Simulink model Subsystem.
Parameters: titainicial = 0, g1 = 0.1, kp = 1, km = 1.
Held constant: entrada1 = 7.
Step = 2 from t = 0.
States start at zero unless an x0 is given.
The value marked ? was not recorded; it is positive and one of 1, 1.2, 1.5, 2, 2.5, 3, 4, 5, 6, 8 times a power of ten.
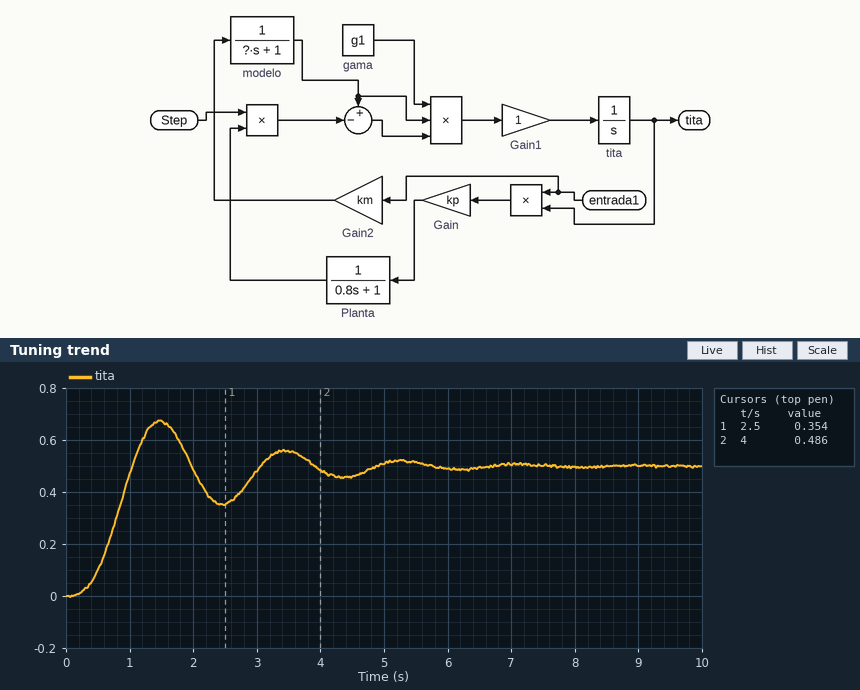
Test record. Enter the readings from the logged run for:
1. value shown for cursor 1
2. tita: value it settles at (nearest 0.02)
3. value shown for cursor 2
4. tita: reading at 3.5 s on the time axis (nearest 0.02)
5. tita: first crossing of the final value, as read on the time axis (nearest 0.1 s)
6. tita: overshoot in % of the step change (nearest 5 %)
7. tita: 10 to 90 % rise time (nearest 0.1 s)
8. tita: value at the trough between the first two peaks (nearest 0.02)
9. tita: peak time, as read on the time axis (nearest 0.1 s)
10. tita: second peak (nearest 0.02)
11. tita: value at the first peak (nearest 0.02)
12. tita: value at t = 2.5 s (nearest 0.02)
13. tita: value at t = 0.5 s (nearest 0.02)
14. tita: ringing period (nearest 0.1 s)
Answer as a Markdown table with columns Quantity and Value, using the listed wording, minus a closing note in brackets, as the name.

| Quantity | Value |
|---|---|
| value shown for cursor 1 | 0.354 |
| tita: value it settles at | 0.50 |
| value shown for cursor 2 | 0.486 |
| tita: reading at 3.5 s on the time axis | 0.56 |
| tita: first crossing of the final value, as read on the time axis | 1.0 s |
| tita: overshoot in % of the step change | 35 % |
| tita: 10 to 90 % rise time | 0.6 s |
| tita: value at the trough between the first two peaks | 0.36 |
| tita: peak time, as read on the time axis | 1.5 s |
| tita: second peak | 0.56 |
| tita: value at the first peak | 0.68 |
| tita: value at t = 2.5 s | 0.36 |
| tita: value at t = 0.5 s | 0.10 |
| tita: ringing period | 2.0 s |
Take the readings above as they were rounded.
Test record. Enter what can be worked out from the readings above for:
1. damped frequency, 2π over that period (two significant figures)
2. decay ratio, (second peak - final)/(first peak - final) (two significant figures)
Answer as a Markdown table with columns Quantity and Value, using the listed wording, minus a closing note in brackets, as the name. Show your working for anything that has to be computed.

| Quantity | Value |
|---|---|
| damped frequency, 2π over that period | 2π / 2 = 3.1 rad/s |
| decay ratio, (second peak - final)/(first peak - final) | (0.56 - 0.5) / (0.68 - 0.5) = 0.33 |
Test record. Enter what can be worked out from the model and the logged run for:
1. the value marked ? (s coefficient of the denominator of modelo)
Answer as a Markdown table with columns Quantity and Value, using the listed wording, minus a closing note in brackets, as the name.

| Quantity | Value |
|---|---|
| the value marked ? | 1.2 |
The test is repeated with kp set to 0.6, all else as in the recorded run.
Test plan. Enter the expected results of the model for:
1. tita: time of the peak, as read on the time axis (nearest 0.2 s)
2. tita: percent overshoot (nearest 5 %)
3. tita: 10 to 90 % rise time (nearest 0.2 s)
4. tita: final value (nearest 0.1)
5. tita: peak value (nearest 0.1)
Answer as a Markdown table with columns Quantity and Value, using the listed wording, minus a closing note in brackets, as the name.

| Quantity | Value |
|---|---|
| tita: time of the peak, as read on the time axis | 1.8 s |
| tita: percent overshoot | 30 % |
| tita: 10 to 90 % rise time | 0.8 s |
| tita: final value | 0.8 |
| tita: peak value | 1.1 |
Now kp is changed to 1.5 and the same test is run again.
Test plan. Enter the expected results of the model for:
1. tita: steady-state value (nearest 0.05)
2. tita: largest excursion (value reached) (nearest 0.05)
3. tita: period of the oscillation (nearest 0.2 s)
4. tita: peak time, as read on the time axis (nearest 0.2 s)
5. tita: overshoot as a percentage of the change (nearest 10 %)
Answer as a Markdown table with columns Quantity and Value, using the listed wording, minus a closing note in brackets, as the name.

| Quantity | Value |
|---|---|
| tita: steady-state value | 0.35 |
| tita: largest excursion (value reached) | 0.45 |
| tita: period of the oscillation | 1.6 s |
| tita: peak time, as read on the time axis | 1.2 s |
| tita: overshoot as a percentage of the change | 40 % |
